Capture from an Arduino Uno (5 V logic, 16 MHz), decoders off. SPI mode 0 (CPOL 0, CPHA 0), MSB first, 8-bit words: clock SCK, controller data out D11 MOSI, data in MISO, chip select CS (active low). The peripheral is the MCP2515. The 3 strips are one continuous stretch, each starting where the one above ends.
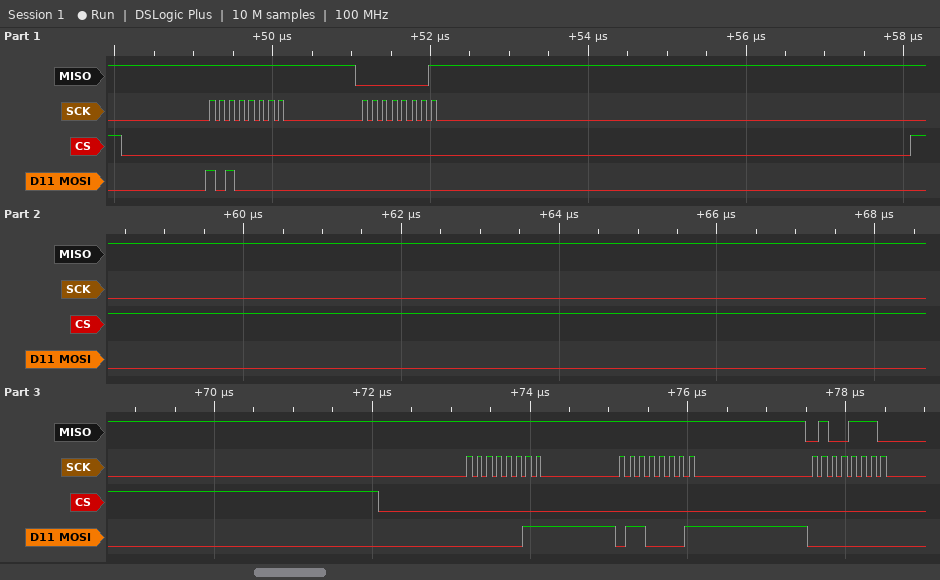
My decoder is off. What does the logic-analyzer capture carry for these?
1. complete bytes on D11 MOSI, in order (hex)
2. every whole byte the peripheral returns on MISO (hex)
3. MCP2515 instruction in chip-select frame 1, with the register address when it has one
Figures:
A0 00 03 61 00
FF 01 FF FF 4E
READ STATUS
